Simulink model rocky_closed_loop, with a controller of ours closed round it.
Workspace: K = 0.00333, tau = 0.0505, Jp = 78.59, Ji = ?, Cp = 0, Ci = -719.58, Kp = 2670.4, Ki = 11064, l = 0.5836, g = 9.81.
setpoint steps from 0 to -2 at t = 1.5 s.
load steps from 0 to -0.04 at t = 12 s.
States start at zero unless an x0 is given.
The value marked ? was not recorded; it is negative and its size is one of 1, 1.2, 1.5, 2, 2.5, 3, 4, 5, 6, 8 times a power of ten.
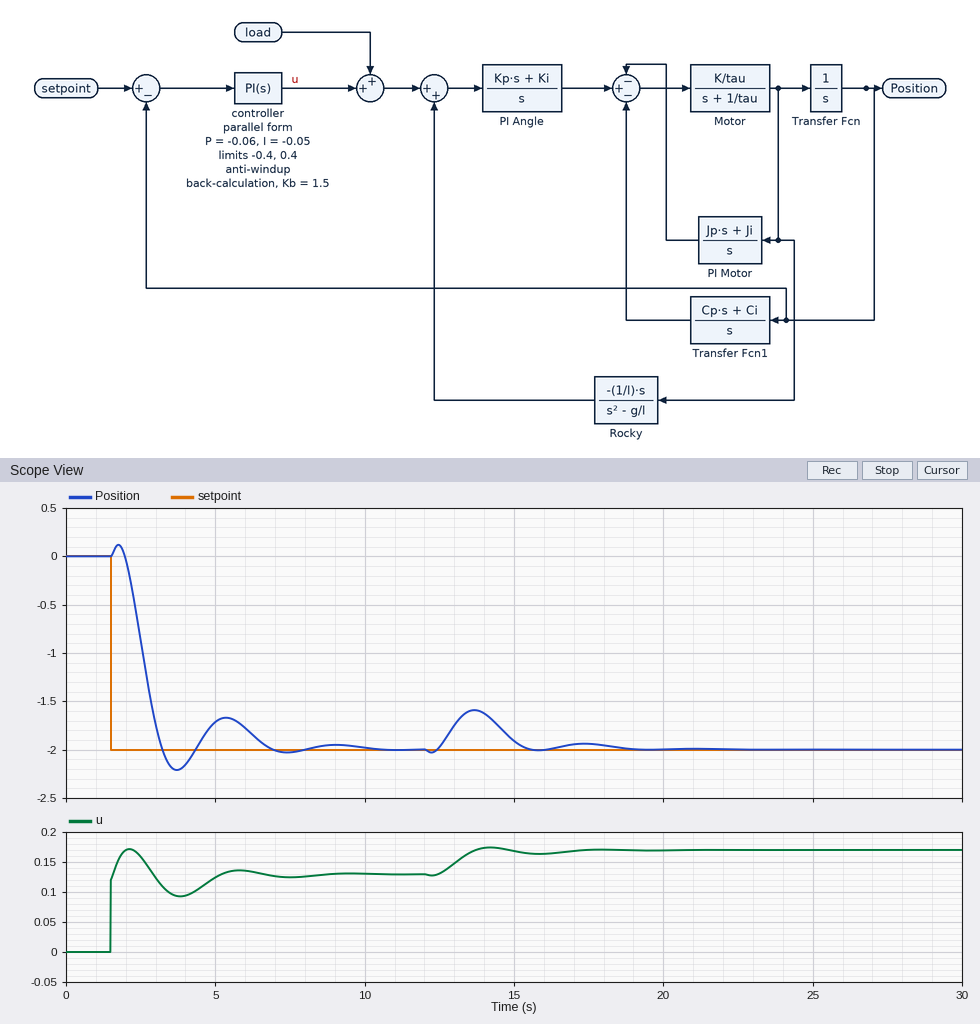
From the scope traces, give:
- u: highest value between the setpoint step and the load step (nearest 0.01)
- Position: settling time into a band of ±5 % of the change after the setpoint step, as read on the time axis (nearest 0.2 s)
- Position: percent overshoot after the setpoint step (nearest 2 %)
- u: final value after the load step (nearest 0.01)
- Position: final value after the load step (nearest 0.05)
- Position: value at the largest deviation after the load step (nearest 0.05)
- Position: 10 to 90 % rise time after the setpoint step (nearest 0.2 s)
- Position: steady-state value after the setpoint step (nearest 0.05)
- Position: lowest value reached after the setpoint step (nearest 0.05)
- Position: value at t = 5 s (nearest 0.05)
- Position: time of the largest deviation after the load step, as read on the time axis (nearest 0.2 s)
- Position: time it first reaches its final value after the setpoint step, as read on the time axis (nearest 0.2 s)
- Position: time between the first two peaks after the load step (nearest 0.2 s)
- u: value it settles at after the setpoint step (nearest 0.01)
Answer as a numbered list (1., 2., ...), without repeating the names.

1. 0.17
2. 6.4 s
3. 10 %
4. 0.17
5. -2.00
6. -1.60
7. 1.0 s
8. -2.00
9. -2.20
10. -1.70
11. 13.6 s
12. 3.2 s
13. 3.6 s
14. 0.13
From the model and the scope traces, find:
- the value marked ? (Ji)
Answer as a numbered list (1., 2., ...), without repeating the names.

1. -1000
